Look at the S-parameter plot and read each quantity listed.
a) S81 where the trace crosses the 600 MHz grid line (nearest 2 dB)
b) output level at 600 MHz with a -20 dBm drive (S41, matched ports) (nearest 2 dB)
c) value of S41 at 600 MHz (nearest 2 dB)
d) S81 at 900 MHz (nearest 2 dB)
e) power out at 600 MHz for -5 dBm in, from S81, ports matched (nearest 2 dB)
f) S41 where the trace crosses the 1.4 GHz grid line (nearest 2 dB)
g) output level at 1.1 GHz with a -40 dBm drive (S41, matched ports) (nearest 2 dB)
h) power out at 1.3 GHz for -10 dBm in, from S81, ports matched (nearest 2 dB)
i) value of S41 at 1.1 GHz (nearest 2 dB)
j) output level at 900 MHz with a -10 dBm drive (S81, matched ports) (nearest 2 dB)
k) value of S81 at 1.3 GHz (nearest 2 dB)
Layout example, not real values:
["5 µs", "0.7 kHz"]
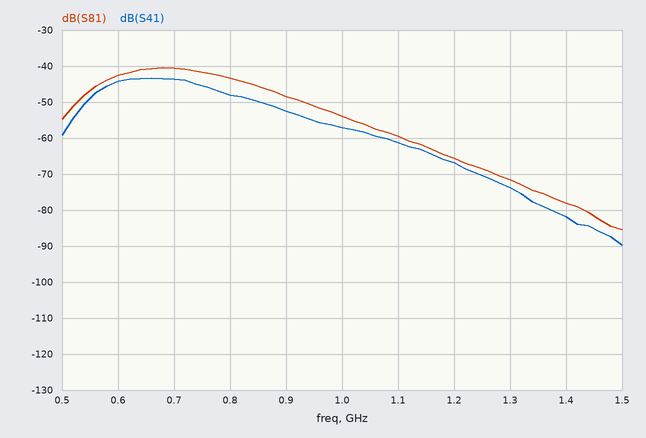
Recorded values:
["-42 dB", "-64 dBm", "-44 dB", "-48 dB", "-48 dBm", "-82 dB", "-102 dBm", "-82 dBm", "-62 dB", "-58 dBm", "-72 dB"]
